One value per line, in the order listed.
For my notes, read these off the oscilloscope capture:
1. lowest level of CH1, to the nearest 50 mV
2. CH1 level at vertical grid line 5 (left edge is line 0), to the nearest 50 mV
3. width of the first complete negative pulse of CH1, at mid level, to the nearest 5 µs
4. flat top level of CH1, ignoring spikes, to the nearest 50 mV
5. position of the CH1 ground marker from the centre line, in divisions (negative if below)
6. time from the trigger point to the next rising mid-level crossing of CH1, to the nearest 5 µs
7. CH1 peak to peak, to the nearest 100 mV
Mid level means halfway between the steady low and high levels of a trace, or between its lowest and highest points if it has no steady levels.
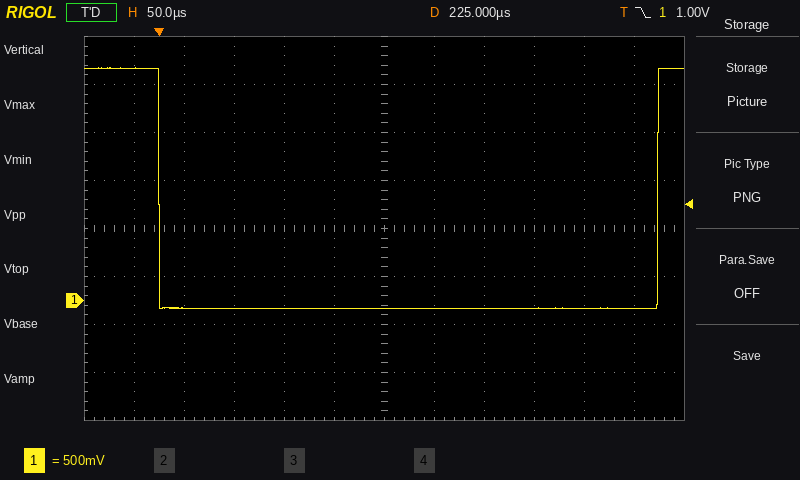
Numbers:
-100 mV
-100 mV
500 µs
2.40 V
-1.5 div
500 µs
2.50 V
